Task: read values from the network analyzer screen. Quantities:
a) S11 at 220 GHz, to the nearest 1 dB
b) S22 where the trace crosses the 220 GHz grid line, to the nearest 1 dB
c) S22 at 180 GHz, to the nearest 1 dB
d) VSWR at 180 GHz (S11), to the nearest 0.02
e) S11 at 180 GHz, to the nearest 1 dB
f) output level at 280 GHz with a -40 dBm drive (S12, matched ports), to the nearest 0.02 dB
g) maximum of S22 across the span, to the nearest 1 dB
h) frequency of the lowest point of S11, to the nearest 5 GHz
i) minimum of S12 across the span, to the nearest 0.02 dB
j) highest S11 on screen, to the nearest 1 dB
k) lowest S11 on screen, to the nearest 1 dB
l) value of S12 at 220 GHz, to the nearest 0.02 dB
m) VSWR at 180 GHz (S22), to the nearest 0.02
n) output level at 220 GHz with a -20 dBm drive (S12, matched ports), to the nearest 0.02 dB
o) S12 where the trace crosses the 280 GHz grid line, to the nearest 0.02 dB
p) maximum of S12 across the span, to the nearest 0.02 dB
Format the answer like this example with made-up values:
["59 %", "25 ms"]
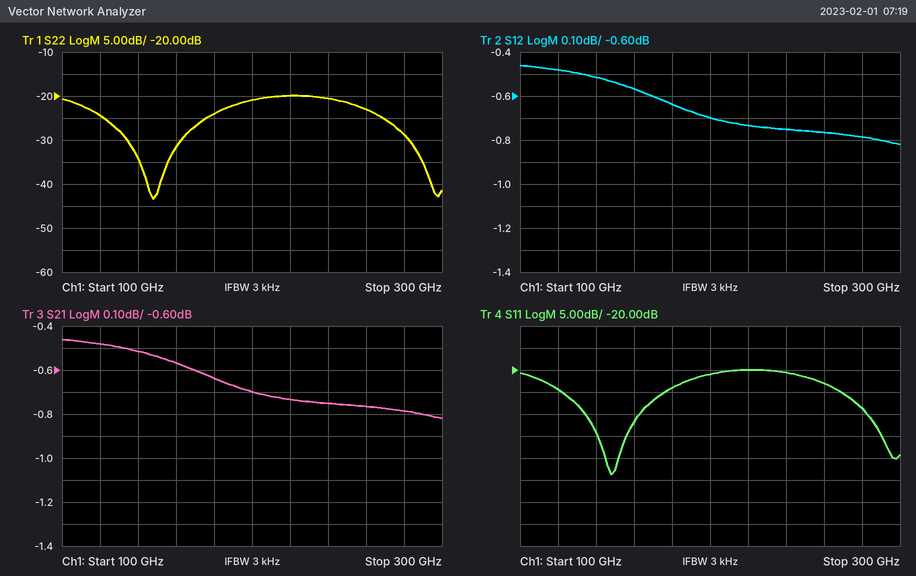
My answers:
["-20 dB", "-20 dB", "-24 dB", "1.14", "-24 dB", "-40.78 dBm", "-20 dB", "150 GHz", "-0.82 dB", "-20 dB", "-44 dB", "-0.74 dB", "1.14", "-20.74 dBm", "-0.78 dB", "-0.46 dB"]
